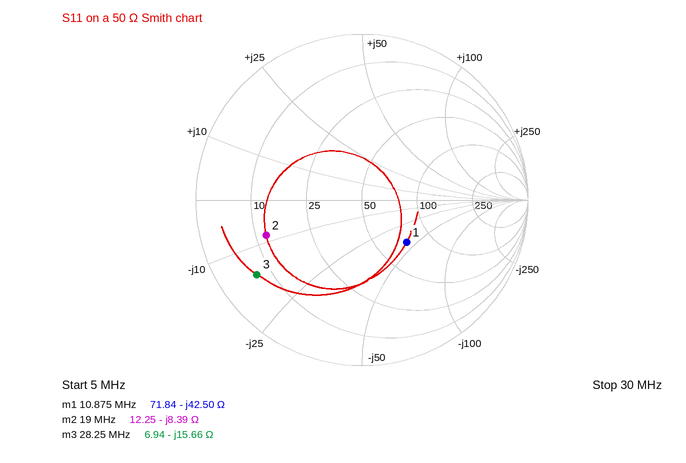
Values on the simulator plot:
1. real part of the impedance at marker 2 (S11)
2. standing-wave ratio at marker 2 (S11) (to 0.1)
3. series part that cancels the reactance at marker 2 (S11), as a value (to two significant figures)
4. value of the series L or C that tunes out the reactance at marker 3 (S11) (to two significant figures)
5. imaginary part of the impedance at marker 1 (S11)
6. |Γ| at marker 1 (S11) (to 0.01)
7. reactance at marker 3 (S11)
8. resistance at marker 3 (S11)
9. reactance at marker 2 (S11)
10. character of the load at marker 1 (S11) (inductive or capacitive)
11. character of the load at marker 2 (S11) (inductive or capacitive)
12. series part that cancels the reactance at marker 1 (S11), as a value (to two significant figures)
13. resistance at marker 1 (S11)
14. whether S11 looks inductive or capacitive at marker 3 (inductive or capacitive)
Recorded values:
12.25 Ω
4.2
70 nH
88 nH
-42.50 Ω
0.37
-15.66 Ω
6.94 Ω
-8.39 Ω
capacitive
capacitive
620 nH
71.84 Ω
capacitive
